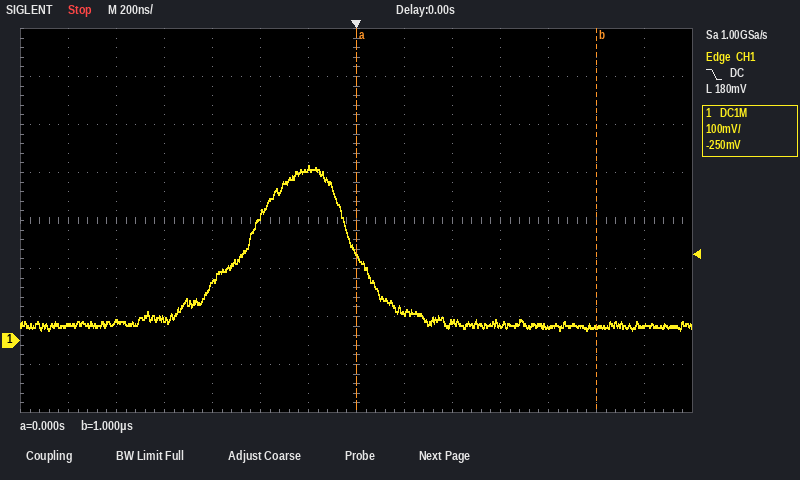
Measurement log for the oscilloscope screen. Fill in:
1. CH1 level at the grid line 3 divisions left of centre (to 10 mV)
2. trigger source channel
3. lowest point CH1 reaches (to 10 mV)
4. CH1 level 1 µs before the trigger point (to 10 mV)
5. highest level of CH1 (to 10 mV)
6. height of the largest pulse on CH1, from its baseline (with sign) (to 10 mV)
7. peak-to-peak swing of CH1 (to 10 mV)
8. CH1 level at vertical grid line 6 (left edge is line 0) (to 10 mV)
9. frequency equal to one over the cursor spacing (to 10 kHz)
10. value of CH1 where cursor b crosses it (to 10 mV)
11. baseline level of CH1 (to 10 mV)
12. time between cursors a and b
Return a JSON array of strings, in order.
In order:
["120 mV", "CH1", "20 mV", "40 mV", "360 mV", "+330 mV", "340 mV", "360 mV", "1.00 MHz", "30 mV", "30 mV", "1.00 µs"]
